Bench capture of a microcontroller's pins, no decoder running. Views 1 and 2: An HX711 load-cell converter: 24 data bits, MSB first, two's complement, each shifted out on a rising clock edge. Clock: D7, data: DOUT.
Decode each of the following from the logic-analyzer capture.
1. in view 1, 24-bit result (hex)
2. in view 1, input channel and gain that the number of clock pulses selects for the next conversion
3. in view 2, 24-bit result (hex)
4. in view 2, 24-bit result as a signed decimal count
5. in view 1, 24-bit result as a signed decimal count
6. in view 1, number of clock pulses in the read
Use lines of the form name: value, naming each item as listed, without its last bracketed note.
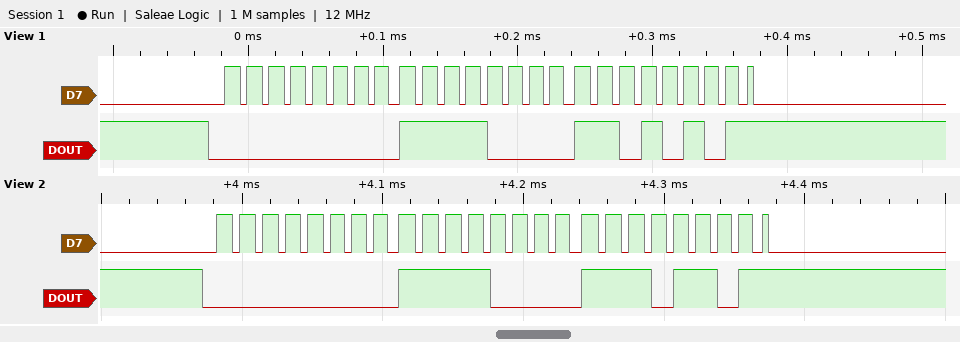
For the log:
in view 1, 24-bit result: 0x00F0D5
in view 1, input channel and gain that the number of clock pulses selects for the next conversion: channel A, gain 128
in view 2, 24-bit result: 0x00F0ED
in view 2, 24-bit result as a signed decimal count: 61677
in view 1, 24-bit result as a signed decimal count: 61653
in view 1, number of clock pulses in the read: 25
